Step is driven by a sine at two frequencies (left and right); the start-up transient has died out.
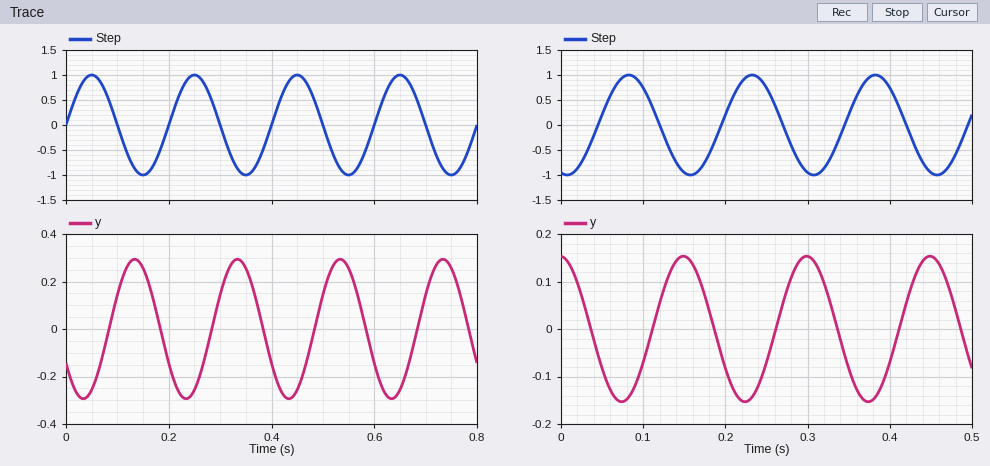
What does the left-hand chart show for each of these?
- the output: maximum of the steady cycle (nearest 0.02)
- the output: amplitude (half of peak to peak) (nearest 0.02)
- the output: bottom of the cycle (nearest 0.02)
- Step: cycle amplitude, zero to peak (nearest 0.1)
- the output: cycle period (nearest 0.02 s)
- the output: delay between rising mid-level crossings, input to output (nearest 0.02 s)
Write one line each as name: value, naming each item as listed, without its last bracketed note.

the output: maximum of the steady cycle: 0.30
the output: amplitude (half of peak to peak): 0.30
the output: bottom of the cycle: -0.30
Step: cycle amplitude, zero to peak: 1.0
the output: cycle period: 0.20 s
the output: delay between rising mid-level crossings, input to output: 0.08 s
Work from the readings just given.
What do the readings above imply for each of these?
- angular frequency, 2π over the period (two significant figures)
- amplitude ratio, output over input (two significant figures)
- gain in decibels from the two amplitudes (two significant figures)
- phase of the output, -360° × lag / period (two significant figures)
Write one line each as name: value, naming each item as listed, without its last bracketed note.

angular frequency, 2π over the period: 31 rad/s
amplitude ratio, output over input: 0.30
gain in decibels from the two amplitudes: -10 dB
phase of the output, -360° × lag / period: -140°
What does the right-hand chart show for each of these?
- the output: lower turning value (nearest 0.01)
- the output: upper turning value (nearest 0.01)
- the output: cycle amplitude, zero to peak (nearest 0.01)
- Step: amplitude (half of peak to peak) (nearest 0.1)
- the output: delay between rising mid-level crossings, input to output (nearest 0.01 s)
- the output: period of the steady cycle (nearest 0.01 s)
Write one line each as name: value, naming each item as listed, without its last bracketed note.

the output: lower turning value: -0.15
the output: upper turning value: 0.15
the output: cycle amplitude, zero to peak: 0.15
Step: amplitude (half of peak to peak): 1.0
the output: delay between rising mid-level crossings, input to output: 0.07 s
the output: period of the steady cycle: 0.15 s
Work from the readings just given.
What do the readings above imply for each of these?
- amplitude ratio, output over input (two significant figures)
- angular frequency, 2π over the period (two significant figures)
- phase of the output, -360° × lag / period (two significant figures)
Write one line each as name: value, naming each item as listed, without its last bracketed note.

amplitude ratio, output over input: 0.15
angular frequency, 2π over the period: 42 rad/s
phase of the output, -360° × lag / period: -170°
